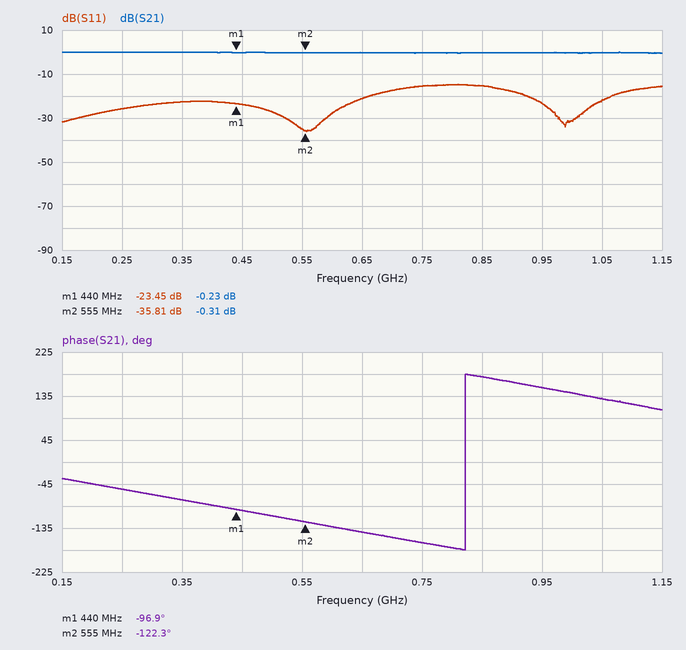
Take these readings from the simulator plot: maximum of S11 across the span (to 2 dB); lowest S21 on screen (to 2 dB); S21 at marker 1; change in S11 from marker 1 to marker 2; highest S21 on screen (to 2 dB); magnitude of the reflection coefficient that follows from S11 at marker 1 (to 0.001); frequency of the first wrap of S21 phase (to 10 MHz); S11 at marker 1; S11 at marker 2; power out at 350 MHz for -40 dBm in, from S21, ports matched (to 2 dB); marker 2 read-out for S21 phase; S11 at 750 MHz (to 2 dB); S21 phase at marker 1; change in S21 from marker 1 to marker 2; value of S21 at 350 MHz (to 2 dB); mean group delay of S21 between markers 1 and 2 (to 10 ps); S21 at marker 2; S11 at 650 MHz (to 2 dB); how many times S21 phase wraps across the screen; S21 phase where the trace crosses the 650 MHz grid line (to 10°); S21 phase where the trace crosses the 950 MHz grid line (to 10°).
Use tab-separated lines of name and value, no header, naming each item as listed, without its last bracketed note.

maximum of S11 across the span	-14 dB
lowest S21 on screen	0 dB
S21 at marker 1	-0.23 dB
change in S11 from marker 1 to marker 2	-12.36 dB
highest S21 on screen	0 dB
magnitude of the reflection coefficient that follows from S11 at marker 1	0.067
frequency of the first wrap of S21 phase	820 MHz
S11 at marker 1	-23.45 dB
S11 at marker 2	-35.81 dB
power out at 350 MHz for -40 dBm in, from S21, ports matched	-40 dBm
marker 2 read-out for S21 phase	-122.3°
S11 at 750 MHz	-16 dB
S21 phase at marker 1	-96.9°
change in S21 from marker 1 to marker 2	-0.08 dB
value of S21 at 350 MHz	0 dB
mean group delay of S21 between markers 1 and 2	610 ps
S21 at marker 2	-0.31 dB
S11 at 650 MHz	-22 dB
how many times S21 phase wraps across the screen	1
S21 phase where the trace crosses the 650 MHz grid line	-140°
S21 phase where the trace crosses the 950 MHz grid line	150°
